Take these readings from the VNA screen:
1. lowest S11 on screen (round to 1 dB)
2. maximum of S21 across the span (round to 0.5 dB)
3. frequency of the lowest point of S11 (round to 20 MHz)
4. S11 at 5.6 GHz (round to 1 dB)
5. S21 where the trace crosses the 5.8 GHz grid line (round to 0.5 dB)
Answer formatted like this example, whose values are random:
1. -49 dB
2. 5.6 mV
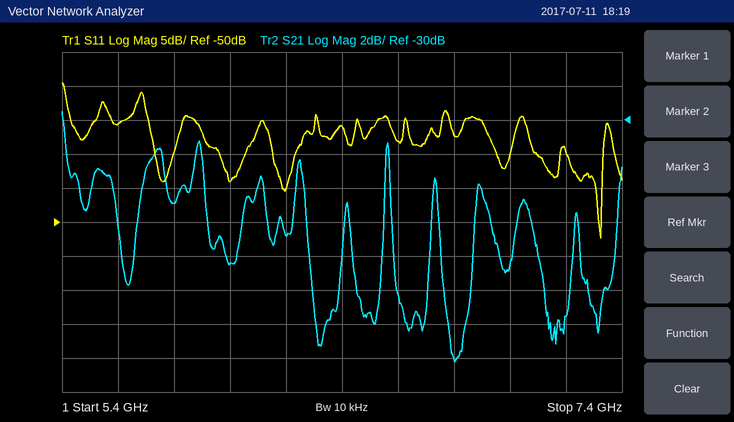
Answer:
1. -52 dB
2. -29.5 dB
3. 7.32 GHz
4. -36 dB
5. -35.0 dB
